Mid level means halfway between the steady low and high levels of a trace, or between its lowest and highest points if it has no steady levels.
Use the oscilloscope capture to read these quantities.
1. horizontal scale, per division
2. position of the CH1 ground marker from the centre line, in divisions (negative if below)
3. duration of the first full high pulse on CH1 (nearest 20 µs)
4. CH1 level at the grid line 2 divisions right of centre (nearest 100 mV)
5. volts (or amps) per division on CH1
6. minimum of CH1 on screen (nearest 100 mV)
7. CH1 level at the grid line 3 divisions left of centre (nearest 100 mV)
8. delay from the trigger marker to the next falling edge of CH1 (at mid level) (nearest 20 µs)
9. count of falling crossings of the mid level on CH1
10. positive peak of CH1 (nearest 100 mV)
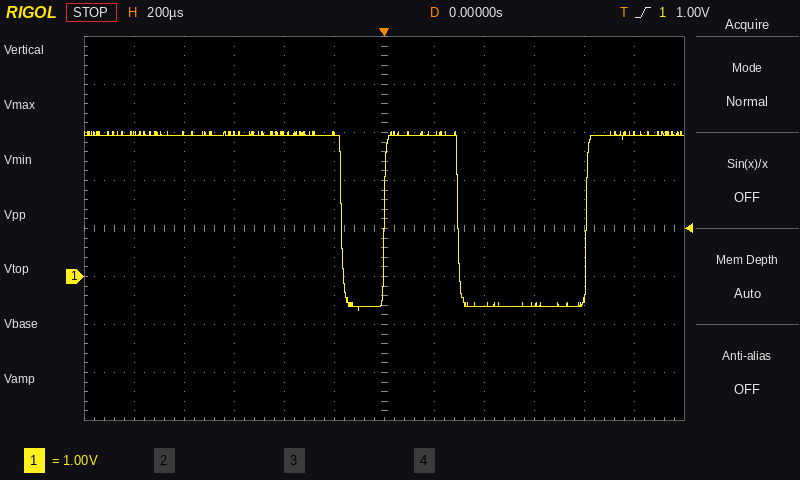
200 µs
-1.0 div
300 µs
-600 mV
1 V
-700 mV
3.0 V
300 µs
2
3.0 V
